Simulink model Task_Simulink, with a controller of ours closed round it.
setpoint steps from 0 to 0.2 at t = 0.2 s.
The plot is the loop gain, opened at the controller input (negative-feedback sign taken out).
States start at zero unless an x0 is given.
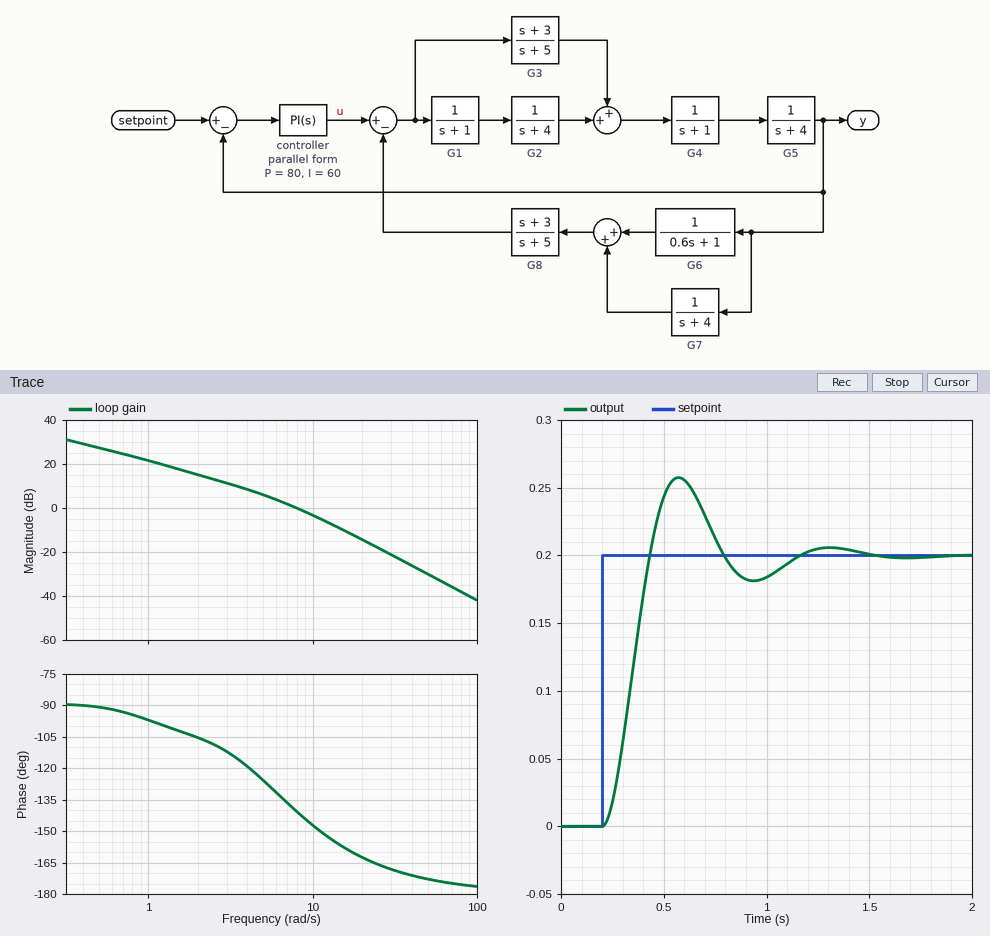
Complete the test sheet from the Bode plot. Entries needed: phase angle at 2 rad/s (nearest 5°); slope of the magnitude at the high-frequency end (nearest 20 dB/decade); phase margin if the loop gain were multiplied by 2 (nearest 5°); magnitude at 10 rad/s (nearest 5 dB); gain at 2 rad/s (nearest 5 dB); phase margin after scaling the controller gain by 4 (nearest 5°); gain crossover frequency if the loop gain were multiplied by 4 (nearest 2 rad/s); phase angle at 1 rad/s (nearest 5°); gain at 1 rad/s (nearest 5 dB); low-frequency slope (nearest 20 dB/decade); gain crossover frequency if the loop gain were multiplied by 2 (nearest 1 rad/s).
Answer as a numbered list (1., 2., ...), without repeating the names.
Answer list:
1. -105°
2. -40 dB/decade
3. 30°
4. -5 dB
5. 15 dB
6. 20°
7. 18 rad/s
8. -95°
9. 20 dB
10. -20 dB/decade
11. 12 rad/s
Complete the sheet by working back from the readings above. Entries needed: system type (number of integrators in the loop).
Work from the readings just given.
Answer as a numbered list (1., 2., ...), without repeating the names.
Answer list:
1. 1
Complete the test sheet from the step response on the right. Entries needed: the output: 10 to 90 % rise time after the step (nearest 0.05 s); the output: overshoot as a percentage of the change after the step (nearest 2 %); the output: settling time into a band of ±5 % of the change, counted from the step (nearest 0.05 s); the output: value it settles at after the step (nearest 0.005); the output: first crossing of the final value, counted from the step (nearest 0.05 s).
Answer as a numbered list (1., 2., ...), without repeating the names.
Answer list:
1. 0.15 s
2. 28 %
3. 0.85 s
4. 0.200
5. 0.25 s
